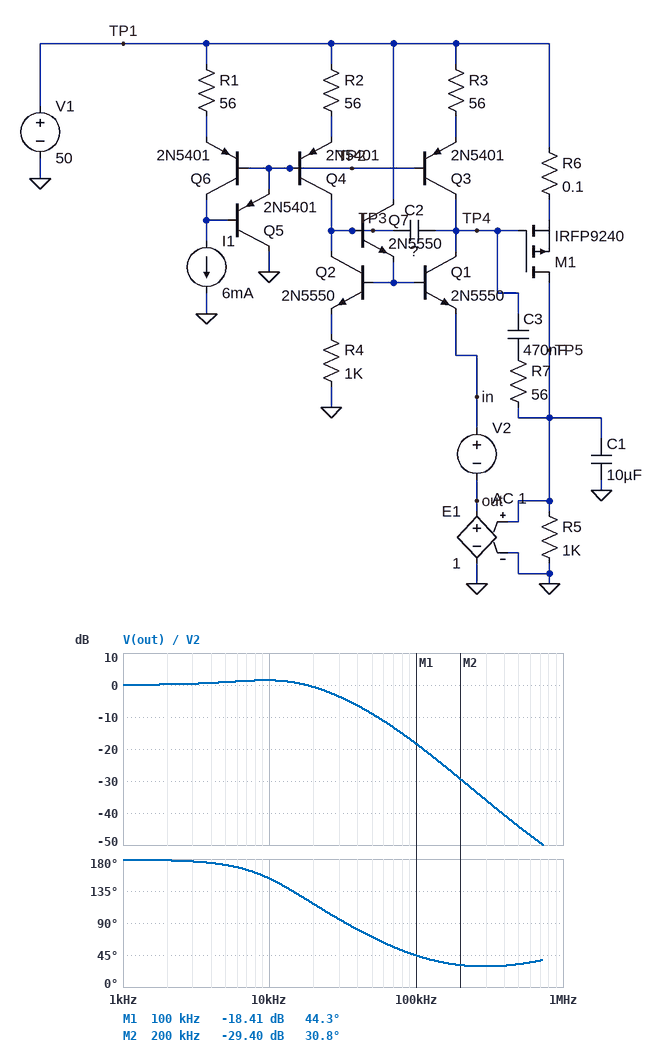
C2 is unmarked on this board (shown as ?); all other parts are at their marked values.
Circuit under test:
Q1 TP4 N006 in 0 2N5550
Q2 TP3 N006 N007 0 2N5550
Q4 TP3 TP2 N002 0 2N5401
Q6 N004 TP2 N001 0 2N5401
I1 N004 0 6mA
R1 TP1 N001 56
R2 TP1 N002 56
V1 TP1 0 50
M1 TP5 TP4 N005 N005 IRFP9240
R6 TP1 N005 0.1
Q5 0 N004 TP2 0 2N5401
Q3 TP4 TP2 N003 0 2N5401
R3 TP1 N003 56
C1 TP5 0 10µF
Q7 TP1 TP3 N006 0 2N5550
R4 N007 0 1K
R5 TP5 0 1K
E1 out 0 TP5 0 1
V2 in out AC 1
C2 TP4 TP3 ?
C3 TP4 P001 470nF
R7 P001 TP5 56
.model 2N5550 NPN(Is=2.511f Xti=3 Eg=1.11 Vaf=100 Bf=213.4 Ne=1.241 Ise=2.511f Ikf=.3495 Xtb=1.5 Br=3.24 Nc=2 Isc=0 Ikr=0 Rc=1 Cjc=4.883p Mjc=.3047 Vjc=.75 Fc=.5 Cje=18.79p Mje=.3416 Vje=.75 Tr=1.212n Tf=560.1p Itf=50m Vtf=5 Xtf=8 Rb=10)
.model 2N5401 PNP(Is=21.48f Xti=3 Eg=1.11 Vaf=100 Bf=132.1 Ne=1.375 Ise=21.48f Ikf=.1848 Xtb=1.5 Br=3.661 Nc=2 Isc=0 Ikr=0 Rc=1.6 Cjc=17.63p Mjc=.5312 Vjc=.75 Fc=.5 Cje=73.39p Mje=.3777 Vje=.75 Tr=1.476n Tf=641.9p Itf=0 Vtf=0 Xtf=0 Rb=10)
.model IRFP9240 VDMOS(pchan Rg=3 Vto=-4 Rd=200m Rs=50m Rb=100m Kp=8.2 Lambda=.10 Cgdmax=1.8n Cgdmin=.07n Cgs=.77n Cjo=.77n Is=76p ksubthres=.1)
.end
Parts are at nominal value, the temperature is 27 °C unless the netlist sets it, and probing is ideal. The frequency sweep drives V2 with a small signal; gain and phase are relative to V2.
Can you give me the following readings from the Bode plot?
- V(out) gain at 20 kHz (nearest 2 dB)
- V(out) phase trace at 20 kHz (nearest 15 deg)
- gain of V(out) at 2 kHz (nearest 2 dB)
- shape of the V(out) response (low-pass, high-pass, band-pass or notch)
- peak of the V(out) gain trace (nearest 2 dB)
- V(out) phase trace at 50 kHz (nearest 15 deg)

0 dB
120 deg
0 dB
low-pass
2 dB
75 deg
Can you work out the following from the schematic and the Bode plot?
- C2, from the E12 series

150 pF
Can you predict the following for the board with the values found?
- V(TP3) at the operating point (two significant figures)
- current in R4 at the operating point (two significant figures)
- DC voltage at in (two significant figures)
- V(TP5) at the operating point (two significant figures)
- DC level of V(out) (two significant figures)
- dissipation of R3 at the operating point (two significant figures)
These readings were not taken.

7.6 V
6.2 mA
6.2 V
6.2 V
6.2 V
2.1 mW
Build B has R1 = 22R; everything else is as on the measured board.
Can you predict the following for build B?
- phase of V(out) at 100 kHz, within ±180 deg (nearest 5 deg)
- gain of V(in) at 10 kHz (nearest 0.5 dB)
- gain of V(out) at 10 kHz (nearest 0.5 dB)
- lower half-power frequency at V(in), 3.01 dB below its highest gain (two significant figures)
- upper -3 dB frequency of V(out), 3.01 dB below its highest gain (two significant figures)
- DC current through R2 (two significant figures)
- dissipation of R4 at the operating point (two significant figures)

55 deg
2.0 dB
-5.0 dB
4.6 kHz
6.9 kHz
2.9 mA
8.5 mW
